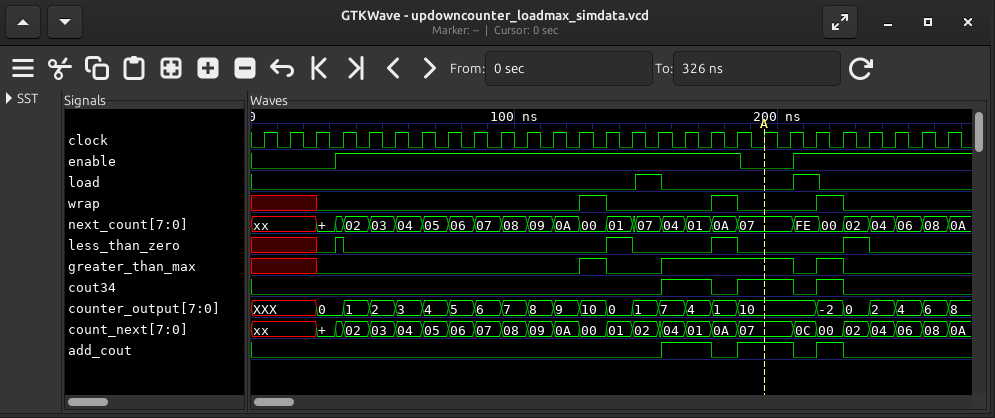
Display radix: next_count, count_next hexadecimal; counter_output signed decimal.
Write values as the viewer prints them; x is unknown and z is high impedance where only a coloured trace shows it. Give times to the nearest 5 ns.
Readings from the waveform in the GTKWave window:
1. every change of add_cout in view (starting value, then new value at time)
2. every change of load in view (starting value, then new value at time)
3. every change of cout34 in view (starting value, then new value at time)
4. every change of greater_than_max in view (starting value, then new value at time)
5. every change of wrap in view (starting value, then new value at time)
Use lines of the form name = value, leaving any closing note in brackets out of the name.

every change of add_cout in view = 0, 1 at 155 ns, 0 at 175 ns, 1 at 185 ns, 0 at 205 ns, 1 at 215 ns, 0 at 225 ns
every change of load in view = 0, 1 at 145 ns, 0 at 155 ns, 1 at 205 ns, 0 at 215 ns
every change of cout34 in view = 0, 1 at 155 ns, 0 at 175 ns, 1 at 185 ns, 0 at 205 ns, 1 at 215 ns, 0 at 225 ns
every change of greater_than_max in view = x, 0 at 25 ns, 1 at 125 ns, 0 at 135 ns, 1 at 155 ns, 0 at 205 ns, 1 at 215 ns, 0 at 225 ns
every change of wrap in view = x, 0 at 25 ns, 1 at 125 ns, 0 at 135 ns, 1 at 175 ns, 0 at 185 ns, 1 at 215 ns, 0 at 225 ns
